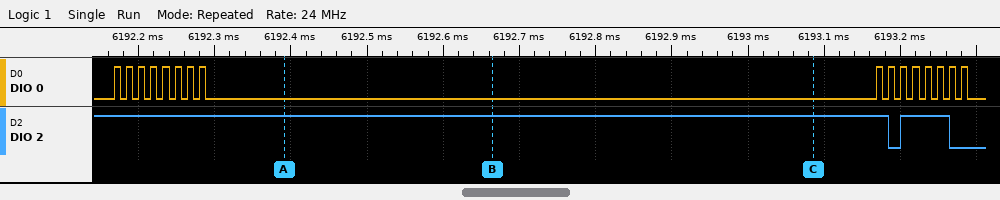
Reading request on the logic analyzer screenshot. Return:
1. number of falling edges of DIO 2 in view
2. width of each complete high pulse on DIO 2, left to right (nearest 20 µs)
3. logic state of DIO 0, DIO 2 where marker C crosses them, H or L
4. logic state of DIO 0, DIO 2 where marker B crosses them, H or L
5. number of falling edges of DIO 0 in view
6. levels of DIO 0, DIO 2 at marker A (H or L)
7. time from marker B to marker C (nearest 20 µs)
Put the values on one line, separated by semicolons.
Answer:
2; 60 µs; DIO 0=L, DIO 2=H; DIO 0=L, DIO 2=H; 16; DIO 0=L, DIO 2=H; 420 µs
